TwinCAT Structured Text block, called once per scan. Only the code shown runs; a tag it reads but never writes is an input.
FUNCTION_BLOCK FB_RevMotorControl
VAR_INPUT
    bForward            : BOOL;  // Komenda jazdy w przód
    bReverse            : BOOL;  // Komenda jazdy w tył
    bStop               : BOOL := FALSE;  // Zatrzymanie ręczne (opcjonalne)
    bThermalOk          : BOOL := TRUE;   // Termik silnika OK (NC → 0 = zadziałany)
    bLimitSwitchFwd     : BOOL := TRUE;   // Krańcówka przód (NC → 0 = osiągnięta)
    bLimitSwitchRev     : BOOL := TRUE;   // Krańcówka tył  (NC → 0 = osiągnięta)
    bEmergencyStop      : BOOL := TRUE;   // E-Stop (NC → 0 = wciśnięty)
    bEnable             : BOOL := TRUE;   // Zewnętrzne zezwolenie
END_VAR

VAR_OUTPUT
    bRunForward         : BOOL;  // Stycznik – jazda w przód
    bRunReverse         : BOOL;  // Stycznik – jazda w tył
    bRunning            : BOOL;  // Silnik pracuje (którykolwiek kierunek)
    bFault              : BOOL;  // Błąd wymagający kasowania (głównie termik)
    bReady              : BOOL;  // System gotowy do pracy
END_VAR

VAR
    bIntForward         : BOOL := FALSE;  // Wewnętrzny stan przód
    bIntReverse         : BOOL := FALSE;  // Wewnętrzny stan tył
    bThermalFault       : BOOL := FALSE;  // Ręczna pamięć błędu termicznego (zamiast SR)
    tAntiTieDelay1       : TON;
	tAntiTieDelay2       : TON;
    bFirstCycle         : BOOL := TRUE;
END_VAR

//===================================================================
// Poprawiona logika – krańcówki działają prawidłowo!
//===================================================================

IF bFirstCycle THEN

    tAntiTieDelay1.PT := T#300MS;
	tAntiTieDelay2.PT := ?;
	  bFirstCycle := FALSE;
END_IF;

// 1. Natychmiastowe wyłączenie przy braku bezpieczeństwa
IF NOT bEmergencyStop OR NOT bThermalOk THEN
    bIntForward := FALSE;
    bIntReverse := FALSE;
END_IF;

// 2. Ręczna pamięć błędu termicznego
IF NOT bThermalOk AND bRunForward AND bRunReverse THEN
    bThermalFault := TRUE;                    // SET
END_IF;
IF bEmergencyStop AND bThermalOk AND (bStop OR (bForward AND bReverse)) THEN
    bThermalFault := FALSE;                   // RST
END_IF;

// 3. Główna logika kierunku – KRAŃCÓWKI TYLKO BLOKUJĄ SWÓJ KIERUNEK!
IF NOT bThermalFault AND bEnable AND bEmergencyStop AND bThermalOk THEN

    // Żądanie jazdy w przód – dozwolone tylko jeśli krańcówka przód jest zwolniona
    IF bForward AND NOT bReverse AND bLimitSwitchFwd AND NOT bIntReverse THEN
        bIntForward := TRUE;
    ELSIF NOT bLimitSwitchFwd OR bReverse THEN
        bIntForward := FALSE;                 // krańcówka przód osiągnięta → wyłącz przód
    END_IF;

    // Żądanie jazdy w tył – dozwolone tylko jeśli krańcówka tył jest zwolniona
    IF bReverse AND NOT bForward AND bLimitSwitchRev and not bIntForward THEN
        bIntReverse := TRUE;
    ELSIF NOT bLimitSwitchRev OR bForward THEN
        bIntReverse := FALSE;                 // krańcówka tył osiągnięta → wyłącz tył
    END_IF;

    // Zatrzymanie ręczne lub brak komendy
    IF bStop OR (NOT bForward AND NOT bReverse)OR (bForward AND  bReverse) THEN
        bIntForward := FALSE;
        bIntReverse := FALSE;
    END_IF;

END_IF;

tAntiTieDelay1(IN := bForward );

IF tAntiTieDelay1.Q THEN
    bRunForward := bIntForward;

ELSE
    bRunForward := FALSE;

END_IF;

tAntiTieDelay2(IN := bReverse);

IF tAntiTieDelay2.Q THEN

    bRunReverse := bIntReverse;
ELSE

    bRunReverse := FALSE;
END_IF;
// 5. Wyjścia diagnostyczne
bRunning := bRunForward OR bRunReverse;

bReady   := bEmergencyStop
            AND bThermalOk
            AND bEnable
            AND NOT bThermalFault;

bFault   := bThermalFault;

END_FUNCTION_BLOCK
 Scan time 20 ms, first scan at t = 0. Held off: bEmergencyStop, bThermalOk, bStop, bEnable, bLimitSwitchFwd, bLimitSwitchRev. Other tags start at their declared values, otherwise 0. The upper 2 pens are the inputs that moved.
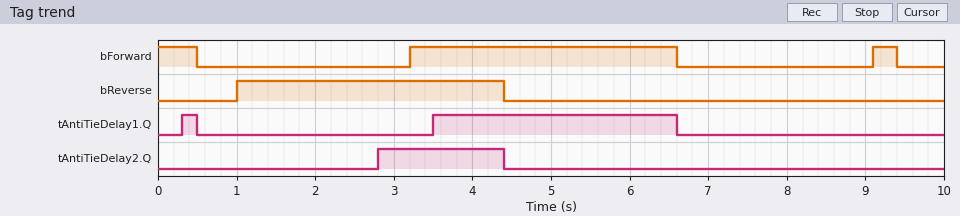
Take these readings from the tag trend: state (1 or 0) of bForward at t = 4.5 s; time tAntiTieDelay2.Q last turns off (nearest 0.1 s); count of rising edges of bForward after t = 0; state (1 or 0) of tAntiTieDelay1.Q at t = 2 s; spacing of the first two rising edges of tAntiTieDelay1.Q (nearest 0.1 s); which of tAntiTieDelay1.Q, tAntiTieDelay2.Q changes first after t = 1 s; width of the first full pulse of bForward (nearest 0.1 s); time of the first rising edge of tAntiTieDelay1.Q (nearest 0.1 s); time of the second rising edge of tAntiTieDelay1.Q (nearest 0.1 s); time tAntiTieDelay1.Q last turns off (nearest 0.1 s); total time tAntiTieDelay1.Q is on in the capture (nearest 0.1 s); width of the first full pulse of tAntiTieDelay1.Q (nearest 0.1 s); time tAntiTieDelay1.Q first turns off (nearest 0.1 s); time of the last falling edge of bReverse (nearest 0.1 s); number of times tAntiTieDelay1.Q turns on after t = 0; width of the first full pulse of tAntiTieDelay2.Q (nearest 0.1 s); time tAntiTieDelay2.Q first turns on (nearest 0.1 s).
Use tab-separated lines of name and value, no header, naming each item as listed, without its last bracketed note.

state (1 or 0) of bForward at t = 4.5 s	1
time tAntiTieDelay2.Q last turns off	4.4 s
count of rising edges of bForward after t = 0	2
state (1 or 0) of tAntiTieDelay1.Q at t = 2 s	0
spacing of the first two rising edges of tAntiTieDelay1.Q	3.2 s
which of tAntiTieDelay1.Q, tAntiTieDelay2.Q changes first after t = 1 s	tAntiTieDelay2.Q
width of the first full pulse of bForward	3.4 s
time of the first rising edge of tAntiTieDelay1.Q	0.3 s
time of the second rising edge of tAntiTieDelay1.Q	3.5 s
time tAntiTieDelay1.Q last turns off	6.6 s
total time tAntiTieDelay1.Q is on in the capture	3.3 s
width of the first full pulse of tAntiTieDelay1.Q	0.2 s
time tAntiTieDelay1.Q first turns off	0.5 s
time of the last falling edge of bReverse	4.4 s
number of times tAntiTieDelay1.Q turns on after t = 0	2
width of the first full pulse of tAntiTieDelay2.Q	1.6 s
time tAntiTieDelay2.Q first turns on	2.8 s
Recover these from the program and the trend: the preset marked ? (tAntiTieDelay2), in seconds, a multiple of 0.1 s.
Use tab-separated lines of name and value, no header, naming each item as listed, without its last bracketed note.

the preset marked ? (tAntiTieDelay2), in seconds, a multiple of 0.1 s	1.8 s
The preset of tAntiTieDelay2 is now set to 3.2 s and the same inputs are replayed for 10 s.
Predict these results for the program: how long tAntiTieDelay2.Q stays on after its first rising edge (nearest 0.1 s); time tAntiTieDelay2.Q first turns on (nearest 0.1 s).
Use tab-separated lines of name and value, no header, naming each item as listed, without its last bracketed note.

how long tAntiTieDelay2.Q stays on after its first rising edge	0.2 s
time tAntiTieDelay2.Q first turns on	4.2 s
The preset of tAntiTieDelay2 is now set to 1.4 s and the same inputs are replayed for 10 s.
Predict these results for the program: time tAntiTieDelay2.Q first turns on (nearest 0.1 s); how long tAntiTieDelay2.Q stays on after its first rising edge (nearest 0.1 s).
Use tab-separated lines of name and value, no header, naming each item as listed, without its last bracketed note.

time tAntiTieDelay2.Q first turns on	2.4 s
how long tAntiTieDelay2.Q stays on after its first rising edge	2.0 s
